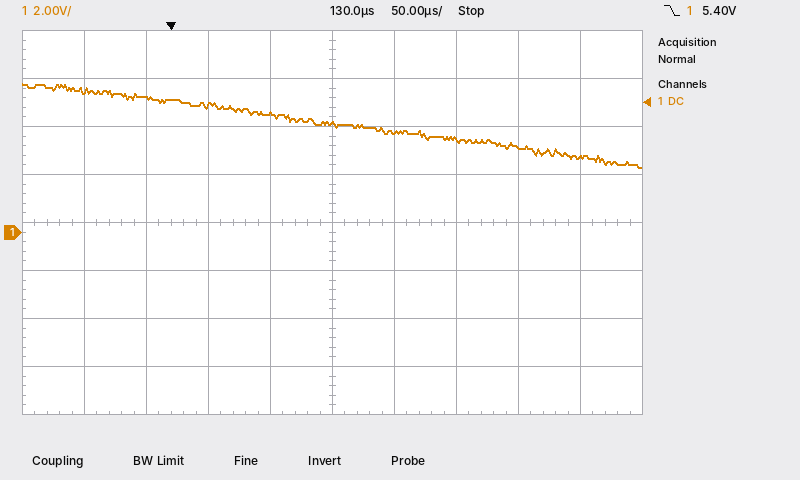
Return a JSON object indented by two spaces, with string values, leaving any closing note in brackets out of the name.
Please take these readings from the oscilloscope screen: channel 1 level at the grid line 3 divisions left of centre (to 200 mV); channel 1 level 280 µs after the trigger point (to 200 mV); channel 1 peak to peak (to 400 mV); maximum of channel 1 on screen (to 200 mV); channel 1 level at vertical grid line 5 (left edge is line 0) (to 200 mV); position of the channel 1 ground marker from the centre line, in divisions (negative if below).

{
  "channel 1 level at the grid line 3 divisions left of centre": "5.6 V",
  "channel 1 level 280 µs after the trigger point": "3.6 V",
  "channel 1 peak to peak": "3.6 V",
  "maximum of channel 1 on screen": "6.2 V",
  "channel 1 level at vertical grid line 5 (left edge is line 0)": "4.6 V",
  "position of the channel 1 ground marker from the centre line, in divisions": "-0.2 div"
}
